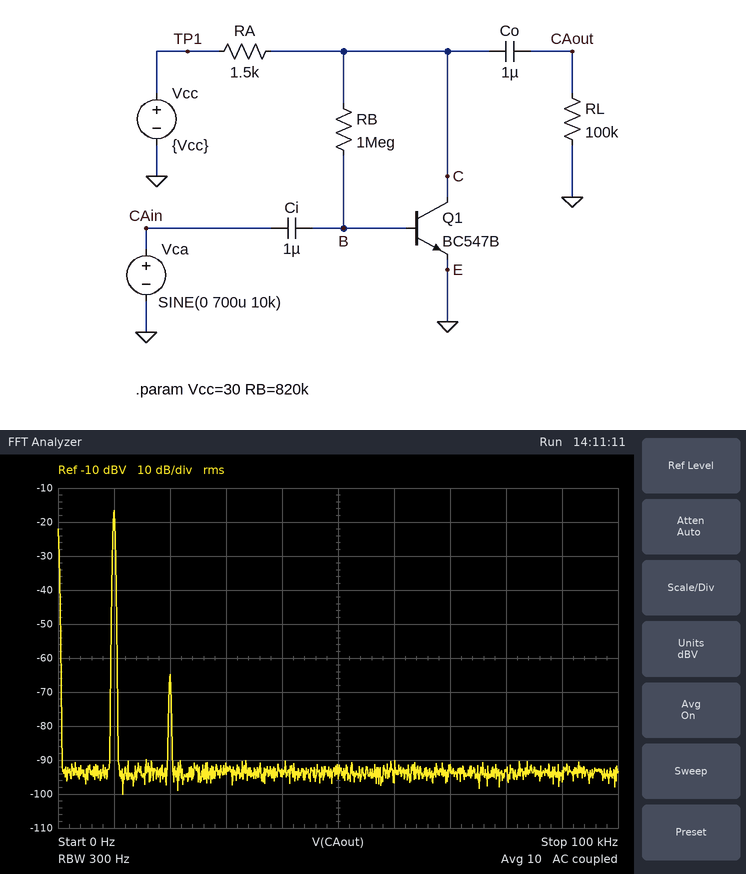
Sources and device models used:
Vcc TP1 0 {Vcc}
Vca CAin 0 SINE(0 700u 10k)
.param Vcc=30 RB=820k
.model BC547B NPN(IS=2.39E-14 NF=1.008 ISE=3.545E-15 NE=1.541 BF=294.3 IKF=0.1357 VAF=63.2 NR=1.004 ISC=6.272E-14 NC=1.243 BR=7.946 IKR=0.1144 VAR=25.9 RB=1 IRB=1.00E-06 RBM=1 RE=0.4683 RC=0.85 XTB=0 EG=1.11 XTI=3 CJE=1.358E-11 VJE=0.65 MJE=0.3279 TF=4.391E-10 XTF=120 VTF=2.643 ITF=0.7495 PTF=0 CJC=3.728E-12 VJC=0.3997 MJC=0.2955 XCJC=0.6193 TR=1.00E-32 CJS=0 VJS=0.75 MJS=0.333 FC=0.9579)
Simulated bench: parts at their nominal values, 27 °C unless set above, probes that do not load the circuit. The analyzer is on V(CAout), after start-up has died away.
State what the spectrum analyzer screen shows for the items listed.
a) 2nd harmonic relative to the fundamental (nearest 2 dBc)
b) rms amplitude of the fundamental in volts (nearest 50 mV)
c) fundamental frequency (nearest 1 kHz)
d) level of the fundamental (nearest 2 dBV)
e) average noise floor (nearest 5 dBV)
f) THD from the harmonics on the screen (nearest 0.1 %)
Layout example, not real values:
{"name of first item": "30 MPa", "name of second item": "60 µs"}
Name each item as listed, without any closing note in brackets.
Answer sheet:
{"2nd harmonic relative to the fundamental": "-48 dBc", "rms amplitude of the fundamental in volts": "150 mV", "fundamental frequency": "10 kHz", "level of the fundamental": "-16 dBV", "average noise floor": "-95 dBV", "THD from the harmonics on the screen": "0.4 %"}
